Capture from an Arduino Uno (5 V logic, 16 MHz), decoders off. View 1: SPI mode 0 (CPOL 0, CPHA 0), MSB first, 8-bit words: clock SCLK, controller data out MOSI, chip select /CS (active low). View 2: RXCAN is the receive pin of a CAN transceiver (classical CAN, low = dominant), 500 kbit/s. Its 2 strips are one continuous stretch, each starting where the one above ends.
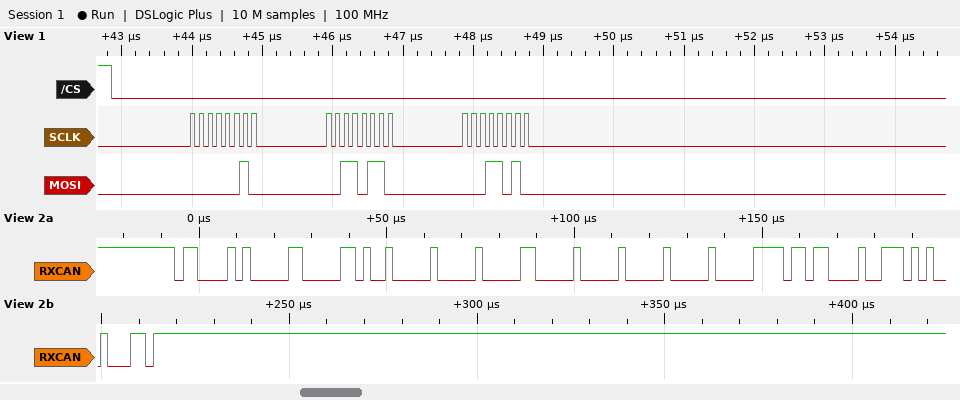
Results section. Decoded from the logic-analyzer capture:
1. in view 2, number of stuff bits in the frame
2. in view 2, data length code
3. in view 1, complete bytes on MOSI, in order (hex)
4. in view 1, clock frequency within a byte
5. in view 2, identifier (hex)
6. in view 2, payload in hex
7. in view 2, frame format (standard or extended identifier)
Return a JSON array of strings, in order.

["10", "8", "02 36 1A", "8 MHz", "0x614", "29 00 01 00 00 00 76 C2", "standard"]
